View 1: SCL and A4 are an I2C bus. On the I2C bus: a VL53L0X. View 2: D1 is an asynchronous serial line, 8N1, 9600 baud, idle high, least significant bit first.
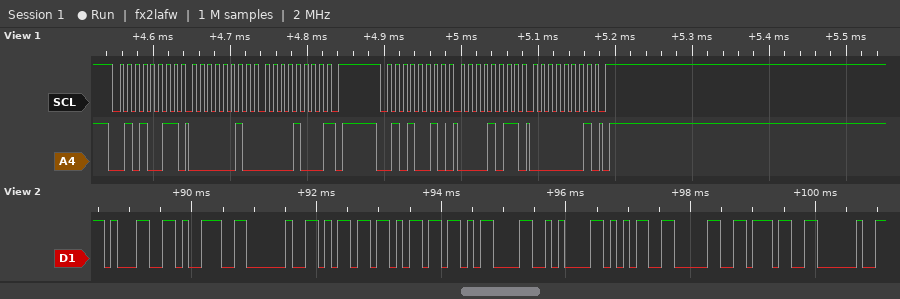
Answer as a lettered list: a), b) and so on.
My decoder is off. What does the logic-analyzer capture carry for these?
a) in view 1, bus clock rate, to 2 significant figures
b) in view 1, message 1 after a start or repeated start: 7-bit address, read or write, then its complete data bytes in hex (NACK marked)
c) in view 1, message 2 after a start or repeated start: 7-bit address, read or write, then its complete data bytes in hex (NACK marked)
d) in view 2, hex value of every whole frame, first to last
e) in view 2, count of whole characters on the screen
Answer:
a) 100 kHz
b) 0x29 read: 02 08 NACK
c) 0x29 write: 0B 01
d) 31 39 20 6D 6D 0D 0A 35 30 37 20
e) 11
